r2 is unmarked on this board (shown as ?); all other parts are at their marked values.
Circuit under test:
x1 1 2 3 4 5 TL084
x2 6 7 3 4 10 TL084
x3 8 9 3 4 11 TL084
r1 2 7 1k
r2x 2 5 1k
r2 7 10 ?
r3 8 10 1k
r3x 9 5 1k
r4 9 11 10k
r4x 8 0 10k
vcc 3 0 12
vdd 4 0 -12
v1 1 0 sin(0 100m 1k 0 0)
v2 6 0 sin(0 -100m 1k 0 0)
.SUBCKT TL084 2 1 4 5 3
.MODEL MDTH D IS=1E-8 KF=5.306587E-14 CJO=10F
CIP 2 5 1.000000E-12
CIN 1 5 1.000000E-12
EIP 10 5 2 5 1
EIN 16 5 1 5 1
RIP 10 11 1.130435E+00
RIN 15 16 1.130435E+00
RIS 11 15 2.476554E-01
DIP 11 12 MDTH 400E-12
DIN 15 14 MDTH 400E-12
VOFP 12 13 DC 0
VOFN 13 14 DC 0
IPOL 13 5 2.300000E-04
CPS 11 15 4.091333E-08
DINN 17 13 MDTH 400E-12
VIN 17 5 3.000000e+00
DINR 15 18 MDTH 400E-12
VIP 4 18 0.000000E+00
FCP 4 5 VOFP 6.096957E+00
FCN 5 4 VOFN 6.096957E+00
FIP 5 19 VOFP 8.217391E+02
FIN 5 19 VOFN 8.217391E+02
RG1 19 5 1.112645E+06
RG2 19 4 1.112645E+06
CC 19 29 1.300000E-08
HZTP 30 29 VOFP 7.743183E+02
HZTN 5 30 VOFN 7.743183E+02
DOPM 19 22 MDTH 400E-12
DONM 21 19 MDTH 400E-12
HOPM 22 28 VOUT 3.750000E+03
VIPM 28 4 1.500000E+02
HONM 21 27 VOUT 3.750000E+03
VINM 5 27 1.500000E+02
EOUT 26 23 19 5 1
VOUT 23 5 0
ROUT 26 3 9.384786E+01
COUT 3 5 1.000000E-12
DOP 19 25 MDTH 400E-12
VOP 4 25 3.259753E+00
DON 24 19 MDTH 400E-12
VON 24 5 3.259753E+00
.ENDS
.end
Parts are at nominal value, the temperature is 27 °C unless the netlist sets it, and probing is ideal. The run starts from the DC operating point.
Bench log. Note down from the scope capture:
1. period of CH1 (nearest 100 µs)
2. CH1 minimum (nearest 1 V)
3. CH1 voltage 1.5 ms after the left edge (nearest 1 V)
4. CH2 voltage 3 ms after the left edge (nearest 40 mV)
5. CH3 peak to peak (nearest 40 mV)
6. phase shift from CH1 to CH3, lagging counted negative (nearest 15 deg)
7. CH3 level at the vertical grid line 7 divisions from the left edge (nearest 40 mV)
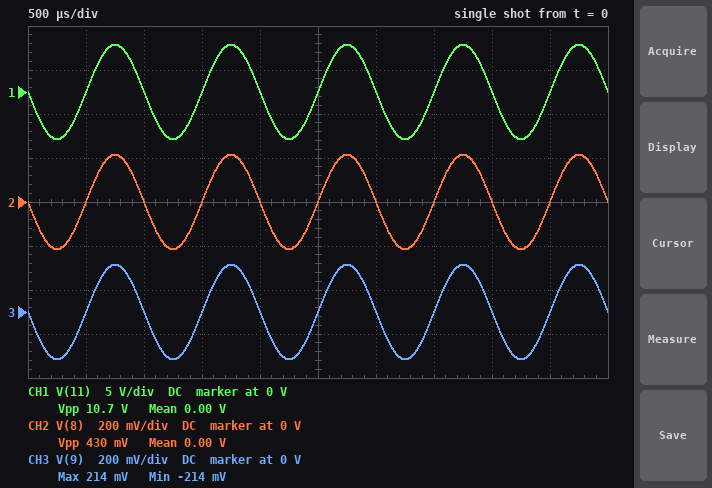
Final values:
1.0 ms
-5 V
0 V
0 V
440 mV
0 deg
0 V
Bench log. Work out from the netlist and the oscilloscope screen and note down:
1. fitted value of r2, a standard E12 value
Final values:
680 Ω
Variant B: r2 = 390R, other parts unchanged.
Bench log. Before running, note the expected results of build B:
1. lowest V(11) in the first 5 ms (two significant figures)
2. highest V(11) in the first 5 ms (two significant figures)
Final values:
-4.8 V
4.8 V
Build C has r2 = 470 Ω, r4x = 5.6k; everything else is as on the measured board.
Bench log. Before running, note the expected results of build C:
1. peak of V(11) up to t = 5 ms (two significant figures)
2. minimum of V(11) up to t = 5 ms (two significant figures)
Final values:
4.8 V
-4.8 V
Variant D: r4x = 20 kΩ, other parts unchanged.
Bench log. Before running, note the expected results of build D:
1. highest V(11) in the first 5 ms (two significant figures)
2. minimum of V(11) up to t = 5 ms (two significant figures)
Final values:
5.5 V
-5.5 V
